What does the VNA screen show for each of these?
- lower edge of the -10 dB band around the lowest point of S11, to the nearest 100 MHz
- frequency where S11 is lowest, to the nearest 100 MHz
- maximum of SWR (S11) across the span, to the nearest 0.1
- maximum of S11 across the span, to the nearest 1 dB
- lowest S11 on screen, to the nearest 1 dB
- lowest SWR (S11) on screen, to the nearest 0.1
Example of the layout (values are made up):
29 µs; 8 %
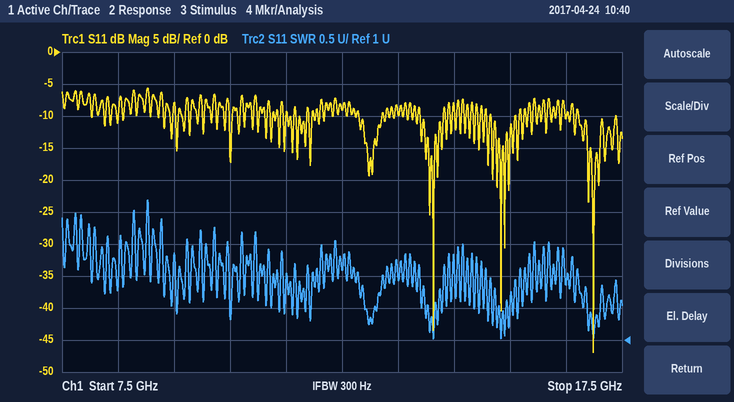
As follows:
16.7 GHz; 17.0 GHz; 3.2; -6 dB; -47 dB; 1.0
